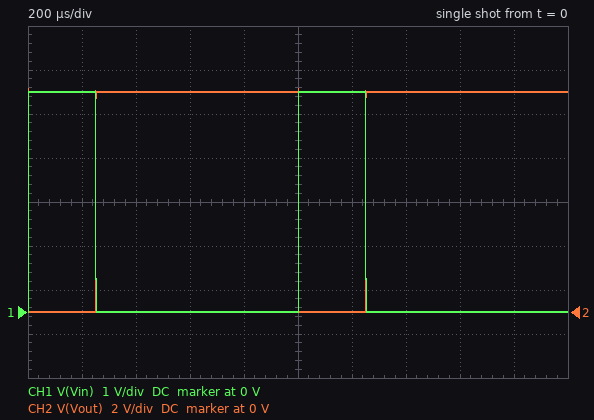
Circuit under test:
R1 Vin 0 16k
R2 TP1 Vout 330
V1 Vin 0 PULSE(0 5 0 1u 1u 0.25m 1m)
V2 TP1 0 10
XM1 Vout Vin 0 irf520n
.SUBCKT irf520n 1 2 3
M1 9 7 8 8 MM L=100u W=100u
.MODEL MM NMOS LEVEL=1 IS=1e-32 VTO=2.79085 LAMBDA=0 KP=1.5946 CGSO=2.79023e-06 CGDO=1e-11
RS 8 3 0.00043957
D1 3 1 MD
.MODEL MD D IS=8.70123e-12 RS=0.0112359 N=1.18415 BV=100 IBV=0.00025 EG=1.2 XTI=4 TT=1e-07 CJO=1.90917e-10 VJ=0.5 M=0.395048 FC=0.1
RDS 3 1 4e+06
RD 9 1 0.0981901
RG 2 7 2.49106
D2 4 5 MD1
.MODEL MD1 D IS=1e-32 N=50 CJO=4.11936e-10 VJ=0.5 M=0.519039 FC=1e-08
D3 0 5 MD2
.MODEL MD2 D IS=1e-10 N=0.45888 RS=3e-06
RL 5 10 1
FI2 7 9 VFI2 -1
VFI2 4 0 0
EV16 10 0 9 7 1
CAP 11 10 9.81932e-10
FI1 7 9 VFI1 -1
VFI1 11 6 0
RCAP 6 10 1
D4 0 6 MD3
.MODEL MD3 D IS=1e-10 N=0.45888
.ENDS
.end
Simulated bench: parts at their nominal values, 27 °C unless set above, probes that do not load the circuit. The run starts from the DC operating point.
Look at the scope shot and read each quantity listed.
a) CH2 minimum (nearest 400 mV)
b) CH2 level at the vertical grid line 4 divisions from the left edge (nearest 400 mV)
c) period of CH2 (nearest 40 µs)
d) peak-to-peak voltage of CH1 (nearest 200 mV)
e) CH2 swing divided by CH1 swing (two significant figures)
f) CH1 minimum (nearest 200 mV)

0 V
10.0 V
1.00 ms
5.0 V
2.0
0 V
